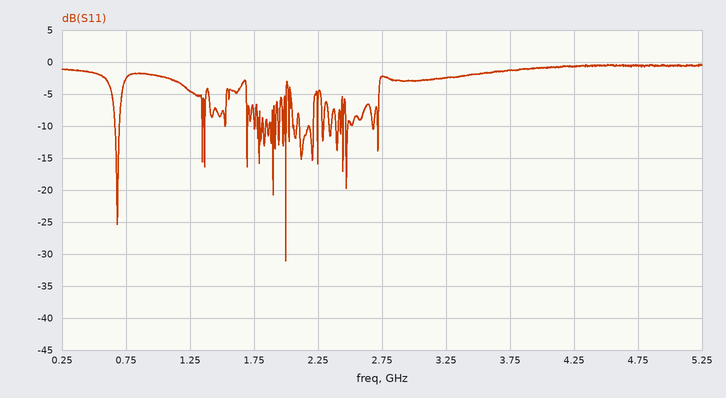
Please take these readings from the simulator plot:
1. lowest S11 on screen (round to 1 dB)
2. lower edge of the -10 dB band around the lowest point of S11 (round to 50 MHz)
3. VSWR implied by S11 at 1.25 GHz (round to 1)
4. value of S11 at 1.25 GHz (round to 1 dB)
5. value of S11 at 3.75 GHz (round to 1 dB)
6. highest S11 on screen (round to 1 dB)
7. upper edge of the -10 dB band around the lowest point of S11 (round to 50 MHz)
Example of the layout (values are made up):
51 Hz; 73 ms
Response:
-31 dB; 2.00 GHz; 4; -5 dB; -1 dB; 0 dB; 2.00 GHz
